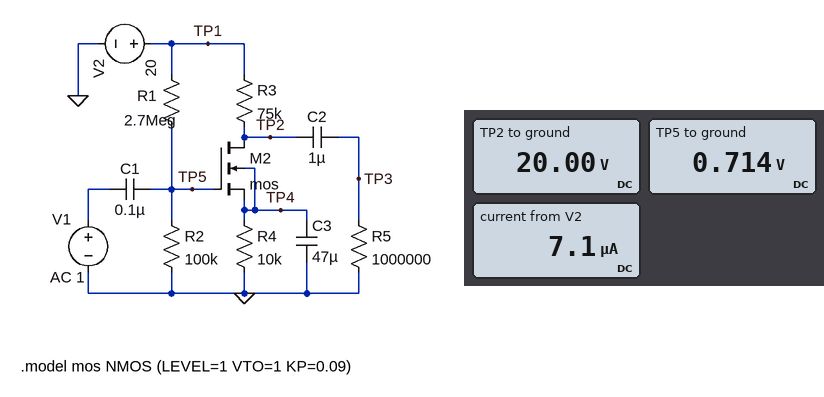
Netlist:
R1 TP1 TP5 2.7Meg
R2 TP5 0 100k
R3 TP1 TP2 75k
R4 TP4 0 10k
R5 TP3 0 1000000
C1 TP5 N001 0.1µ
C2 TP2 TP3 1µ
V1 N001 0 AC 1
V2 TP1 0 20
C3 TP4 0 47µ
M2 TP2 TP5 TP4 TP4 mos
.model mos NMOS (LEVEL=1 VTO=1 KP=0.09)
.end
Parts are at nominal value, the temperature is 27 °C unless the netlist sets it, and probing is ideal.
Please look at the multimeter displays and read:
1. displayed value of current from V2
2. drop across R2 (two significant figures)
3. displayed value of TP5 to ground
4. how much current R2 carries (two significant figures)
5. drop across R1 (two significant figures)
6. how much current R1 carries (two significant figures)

7.1 µA
710 mV
0.714 V
7.1 µA
19 V
7.1 µA
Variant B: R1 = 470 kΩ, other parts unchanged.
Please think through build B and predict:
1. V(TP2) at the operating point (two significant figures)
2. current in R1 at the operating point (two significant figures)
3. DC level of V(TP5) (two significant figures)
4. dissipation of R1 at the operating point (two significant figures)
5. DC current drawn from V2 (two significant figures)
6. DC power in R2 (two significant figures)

2.4 V
35 µA
3.5 V
580 µW
270 µA
120 µW
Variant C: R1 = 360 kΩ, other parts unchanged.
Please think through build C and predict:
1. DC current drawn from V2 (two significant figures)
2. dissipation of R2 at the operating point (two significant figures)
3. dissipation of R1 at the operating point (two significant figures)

280 µA
190 µW
680 µW
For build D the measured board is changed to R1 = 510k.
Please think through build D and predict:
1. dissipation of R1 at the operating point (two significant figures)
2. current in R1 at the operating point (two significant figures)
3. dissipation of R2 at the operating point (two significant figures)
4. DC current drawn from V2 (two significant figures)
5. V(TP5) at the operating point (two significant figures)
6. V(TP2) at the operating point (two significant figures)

550 µW
33 µA
110 µW
250 µA
3.3 V
3.4 V
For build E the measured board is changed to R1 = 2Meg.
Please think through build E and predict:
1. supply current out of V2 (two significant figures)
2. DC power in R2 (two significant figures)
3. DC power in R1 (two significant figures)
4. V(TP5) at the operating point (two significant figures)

9.5 µA
9.1 µW
180 µW
950 mV
